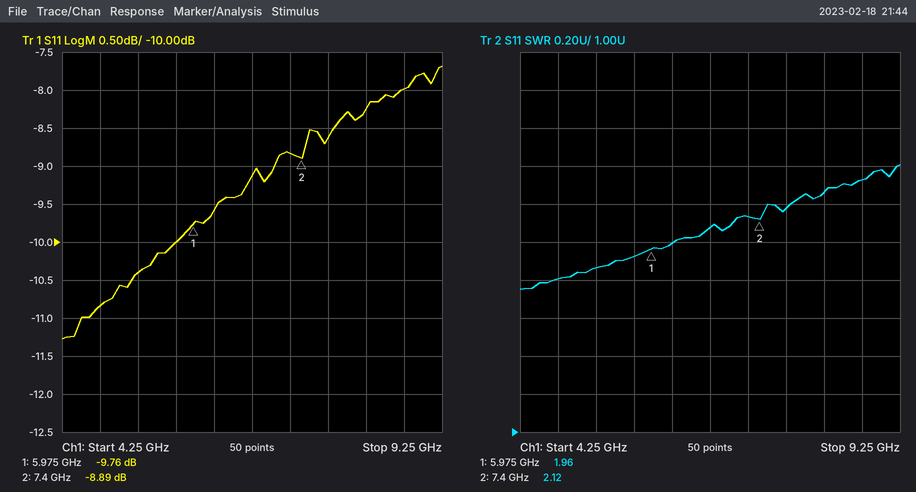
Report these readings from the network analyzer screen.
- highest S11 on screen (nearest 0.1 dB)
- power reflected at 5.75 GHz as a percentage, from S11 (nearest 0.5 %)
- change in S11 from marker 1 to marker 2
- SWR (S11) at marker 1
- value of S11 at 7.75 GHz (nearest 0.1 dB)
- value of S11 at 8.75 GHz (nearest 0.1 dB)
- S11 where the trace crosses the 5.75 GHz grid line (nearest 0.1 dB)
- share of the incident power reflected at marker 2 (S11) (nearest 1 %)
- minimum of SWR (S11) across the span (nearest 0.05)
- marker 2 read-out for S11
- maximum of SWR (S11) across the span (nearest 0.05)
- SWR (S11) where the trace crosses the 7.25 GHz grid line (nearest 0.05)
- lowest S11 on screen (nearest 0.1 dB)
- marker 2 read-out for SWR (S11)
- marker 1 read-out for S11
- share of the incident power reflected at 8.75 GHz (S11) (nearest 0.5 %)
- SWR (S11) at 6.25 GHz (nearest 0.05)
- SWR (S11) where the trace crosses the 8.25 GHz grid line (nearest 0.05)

-7.7 dB
10.0 %
0.87 dB
1.96
-8.6 dB
-8.0 dB
-10.0 dB
13 %
1.75
-8.89 dB
2.40
2.15
-11.3 dB
2.12
-9.76 dB
16.0 %
2.00
2.25
